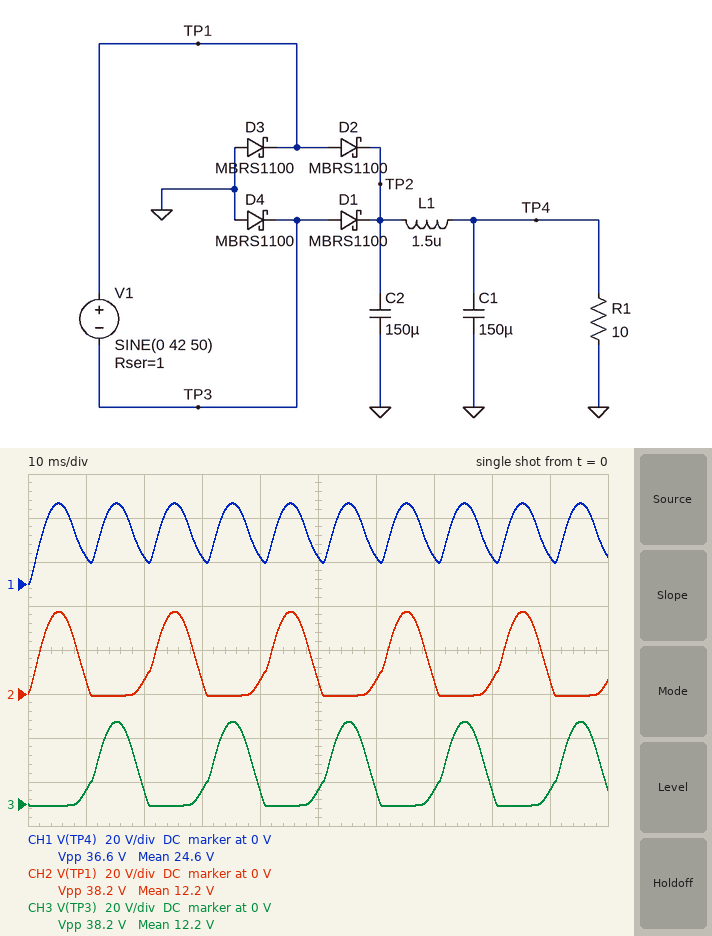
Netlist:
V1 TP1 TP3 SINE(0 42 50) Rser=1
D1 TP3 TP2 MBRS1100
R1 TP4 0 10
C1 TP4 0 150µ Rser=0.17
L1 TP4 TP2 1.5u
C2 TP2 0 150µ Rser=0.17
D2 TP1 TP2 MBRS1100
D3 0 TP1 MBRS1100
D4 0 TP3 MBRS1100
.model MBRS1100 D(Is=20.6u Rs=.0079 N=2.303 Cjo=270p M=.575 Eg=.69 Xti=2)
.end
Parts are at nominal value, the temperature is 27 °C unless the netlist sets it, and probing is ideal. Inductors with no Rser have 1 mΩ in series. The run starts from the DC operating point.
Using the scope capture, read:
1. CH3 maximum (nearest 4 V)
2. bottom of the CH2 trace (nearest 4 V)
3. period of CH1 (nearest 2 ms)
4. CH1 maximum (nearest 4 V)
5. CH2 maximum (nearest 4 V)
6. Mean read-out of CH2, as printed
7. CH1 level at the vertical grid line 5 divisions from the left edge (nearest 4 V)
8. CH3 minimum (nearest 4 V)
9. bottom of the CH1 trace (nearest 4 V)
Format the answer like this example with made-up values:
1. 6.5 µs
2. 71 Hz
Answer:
1. 36 V
2. 0 V
3. 10 ms
4. 36 V
5. 36 V
6. 12.2 V
7. 12 V
8. 0 V
9. 0 V
